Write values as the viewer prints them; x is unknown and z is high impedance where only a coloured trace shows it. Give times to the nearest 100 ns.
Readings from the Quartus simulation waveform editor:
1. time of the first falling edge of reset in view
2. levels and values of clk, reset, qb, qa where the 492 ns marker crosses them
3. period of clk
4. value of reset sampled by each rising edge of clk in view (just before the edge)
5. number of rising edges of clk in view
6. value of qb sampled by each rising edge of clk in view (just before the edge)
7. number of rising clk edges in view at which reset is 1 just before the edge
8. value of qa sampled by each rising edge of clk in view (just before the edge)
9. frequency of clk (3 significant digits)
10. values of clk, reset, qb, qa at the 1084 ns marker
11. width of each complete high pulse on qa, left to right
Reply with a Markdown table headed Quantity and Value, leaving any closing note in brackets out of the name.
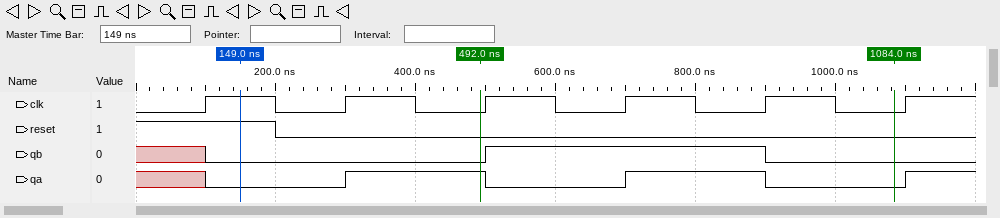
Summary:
| Quantity | Value |
|---|---|
| time of the first falling edge of reset in view | 200 ns |
| levels and values of clk, reset, qb, qa where the 492 ns marker crosses them | clk=0, reset=0, qb=0, qa=1 |
| period of clk | 200 ns |
| value of reset sampled by each rising edge of clk in view | 1 0 0 0 0 0 |
| number of rising edges of clk in view | 6 |
| value of qb sampled by each rising edge of clk in view | x 0 0 1 1 0 |
| number of rising clk edges in view at which reset is 1 just before the edge | 1 |
| value of qa sampled by each rising edge of clk in view | x 0 1 0 1 0 |
| frequency of clk | 5.00 MHz |
| values of clk, reset, qb, qa at the 1084 ns marker | clk=0, reset=0, qb=0, qa=0 |
| width of each complete high pulse on qa, left to right | 200 ns, 200 ns |
